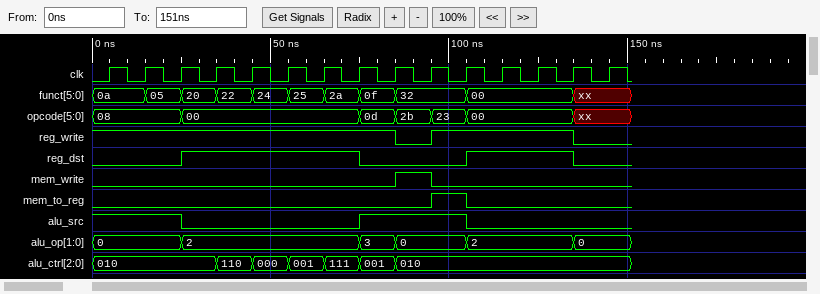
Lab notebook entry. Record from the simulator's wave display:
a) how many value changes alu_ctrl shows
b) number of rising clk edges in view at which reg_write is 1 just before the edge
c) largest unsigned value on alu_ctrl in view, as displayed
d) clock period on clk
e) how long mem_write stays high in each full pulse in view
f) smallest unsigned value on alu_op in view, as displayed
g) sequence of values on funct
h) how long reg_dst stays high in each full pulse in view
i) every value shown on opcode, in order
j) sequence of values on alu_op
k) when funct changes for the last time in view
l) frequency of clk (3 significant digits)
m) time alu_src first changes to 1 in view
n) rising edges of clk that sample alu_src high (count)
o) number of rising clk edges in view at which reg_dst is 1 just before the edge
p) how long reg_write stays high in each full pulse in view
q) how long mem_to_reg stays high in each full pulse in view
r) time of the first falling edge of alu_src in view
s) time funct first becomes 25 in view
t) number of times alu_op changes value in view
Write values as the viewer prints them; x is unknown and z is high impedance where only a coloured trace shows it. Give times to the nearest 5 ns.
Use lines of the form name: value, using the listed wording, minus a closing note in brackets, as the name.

how many value changes alu_ctrl shows: 6
number of rising clk edges in view at which reg_write is 1 just before the edge: 13
largest unsigned value on alu_ctrl in view, as displayed: 111
clock period on clk: 10 ns
how long mem_write stays high in each full pulse in view: 10 ns
smallest unsigned value on alu_op in view, as displayed: 0
sequence of values on funct: 0a, 05, 20, 22, 24, 25, 2a, 0f, 32, 00, xx
how long reg_dst stays high in each full pulse in view: 50 ns, 30 ns
every value shown on opcode, in order: 08, 00, 0d, 2b, 23, 00, xx
sequence of values on alu_op: 0, 2, 3, 0, 2, 0
when funct changes for the last time in view: 135 ns
frequency of clk: 100 MHz
time alu_src first changes to 1 in view: 75 ns
rising edges of clk that sample alu_src high: 6
number of rising clk edges in view at which reg_dst is 1 just before the edge: 8
how long reg_write stays high in each full pulse in view: 40 ns
how long mem_to_reg stays high in each full pulse in view: 10 ns
time of the first falling edge of alu_src in view: 25 ns
time funct first becomes 25 in view: 55 ns
number of times alu_op changes value in view: 5
